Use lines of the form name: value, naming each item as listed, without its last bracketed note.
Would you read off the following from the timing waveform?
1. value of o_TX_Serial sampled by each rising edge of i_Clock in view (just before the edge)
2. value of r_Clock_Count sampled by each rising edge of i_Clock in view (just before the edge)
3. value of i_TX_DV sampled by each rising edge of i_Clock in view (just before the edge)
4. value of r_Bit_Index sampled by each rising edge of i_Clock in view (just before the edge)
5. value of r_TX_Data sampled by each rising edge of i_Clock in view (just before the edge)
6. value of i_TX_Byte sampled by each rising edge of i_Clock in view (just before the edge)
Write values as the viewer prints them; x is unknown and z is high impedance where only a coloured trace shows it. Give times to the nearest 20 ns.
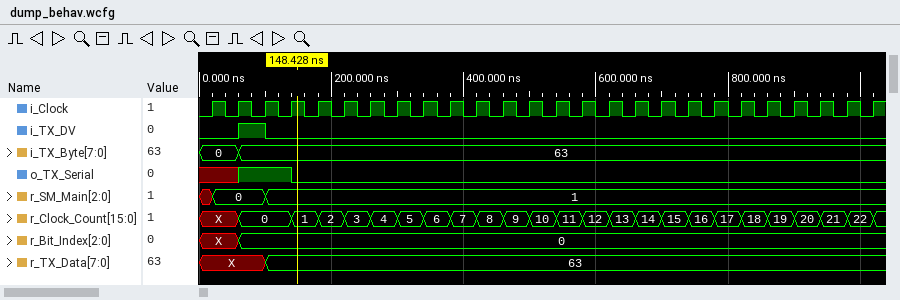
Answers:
value of o_TX_Serial sampled by each rising edge of i_Clock in view: x x 1 1 0 0 0 0 0 0 0 0 0 0 0 0 0 0 0 0 0 0 0 0 0 0
value of r_Clock_Count sampled by each rising edge of i_Clock in view: X, X, 0, 0, 1, 2, 3, 4, 5, 6, 7, 8, 9, 10, 11, 12, 13, 14, 15, 16, 17, 18, 19, 20, 21, 22
value of i_TX_DV sampled by each rising edge of i_Clock in view: 0 0 1 0 0 0 0 0 0 0 0 0 0 0 0 0 0 0 0 0 0 0 0 0 0 0
value of r_Bit_Index sampled by each rising edge of i_Clock in view: X, X, 0, 0, 0, 0, 0, 0, 0, 0, 0, 0, 0, 0, 0, 0, 0, 0, 0, 0, 0, 0, 0, 0, 0, 0
value of r_TX_Data sampled by each rising edge of i_Clock in view: X, X, X, 63, 63, 63, 63, 63, 63, 63, 63, 63, 63, 63, 63, 63, 63, 63, 63, 63, 63, 63, 63, 63, 63, 63
value of i_TX_Byte sampled by each rising edge of i_Clock in view: 0, 0, 63, 63, 63, 63, 63, 63, 63, 63, 63, 63, 63, 63, 63, 63, 63, 63, 63, 63, 63, 63, 63, 63, 63, 63
